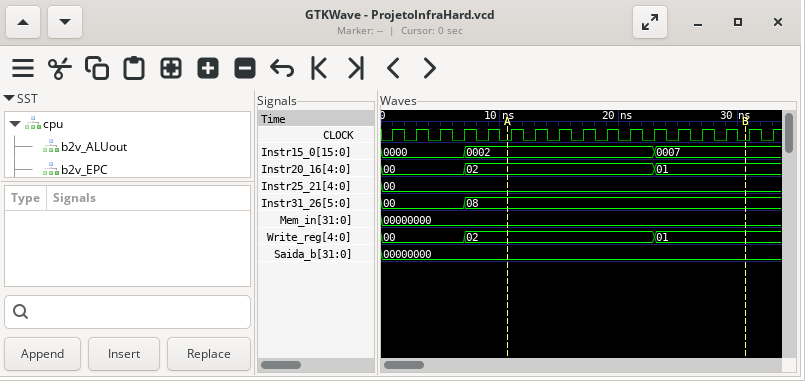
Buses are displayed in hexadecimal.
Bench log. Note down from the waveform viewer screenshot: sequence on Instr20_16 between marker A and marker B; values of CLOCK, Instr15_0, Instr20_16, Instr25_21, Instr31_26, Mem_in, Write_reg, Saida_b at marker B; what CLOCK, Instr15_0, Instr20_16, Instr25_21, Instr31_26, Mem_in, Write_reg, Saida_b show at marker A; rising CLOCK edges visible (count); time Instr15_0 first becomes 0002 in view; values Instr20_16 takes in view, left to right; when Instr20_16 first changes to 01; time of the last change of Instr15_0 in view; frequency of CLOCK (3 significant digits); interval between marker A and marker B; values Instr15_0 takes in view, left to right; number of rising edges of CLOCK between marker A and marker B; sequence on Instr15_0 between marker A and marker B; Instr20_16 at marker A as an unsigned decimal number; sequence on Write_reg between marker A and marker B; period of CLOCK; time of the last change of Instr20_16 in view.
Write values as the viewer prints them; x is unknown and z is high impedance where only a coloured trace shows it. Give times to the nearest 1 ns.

02, 01
CLOCK=0, Instr15_0=0007, Instr20_16=01, Instr25_21=00, Instr31_26=08, Mem_in=00000000, Write_reg=01, Saida_b=00000000
CLOCK=0, Instr15_0=0002, Instr20_16=02, Instr25_21=00, Instr31_26=08, Mem_in=00000000, Write_reg=02, Saida_b=00000000
17
7 ns
00, 02, 01
23 ns
23 ns
500 MHz
20 ns
0000, 0002, 0007
10
0002, 0007
2
02, 01
2 ns
23 ns
